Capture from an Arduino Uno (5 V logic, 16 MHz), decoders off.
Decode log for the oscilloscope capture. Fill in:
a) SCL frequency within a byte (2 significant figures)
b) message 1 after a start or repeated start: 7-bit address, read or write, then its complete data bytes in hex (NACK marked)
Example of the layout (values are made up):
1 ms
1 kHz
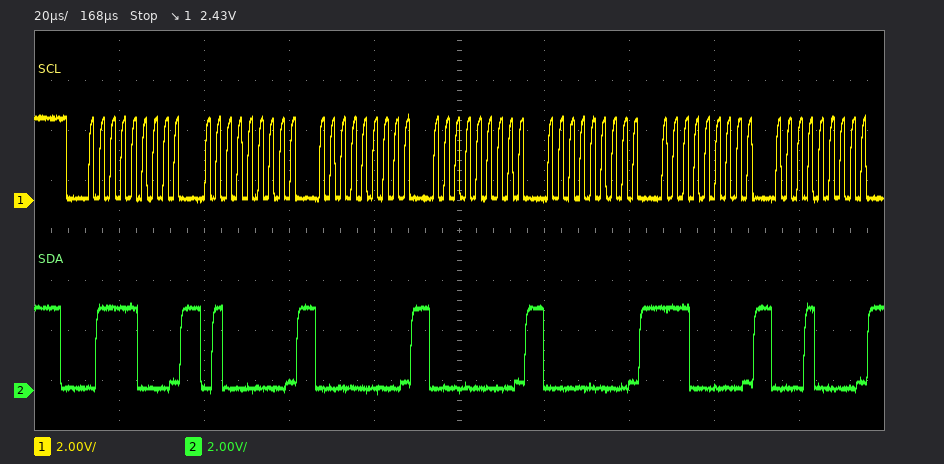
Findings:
400 kHz
0x3C write: 40 00 00 00 E0 10
